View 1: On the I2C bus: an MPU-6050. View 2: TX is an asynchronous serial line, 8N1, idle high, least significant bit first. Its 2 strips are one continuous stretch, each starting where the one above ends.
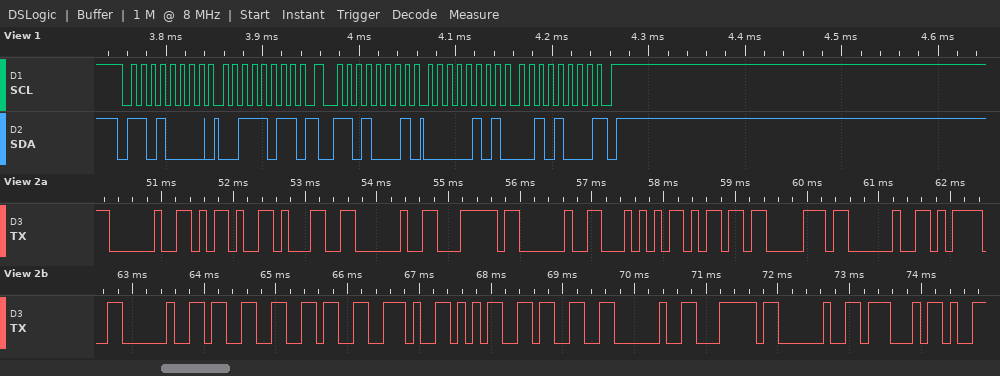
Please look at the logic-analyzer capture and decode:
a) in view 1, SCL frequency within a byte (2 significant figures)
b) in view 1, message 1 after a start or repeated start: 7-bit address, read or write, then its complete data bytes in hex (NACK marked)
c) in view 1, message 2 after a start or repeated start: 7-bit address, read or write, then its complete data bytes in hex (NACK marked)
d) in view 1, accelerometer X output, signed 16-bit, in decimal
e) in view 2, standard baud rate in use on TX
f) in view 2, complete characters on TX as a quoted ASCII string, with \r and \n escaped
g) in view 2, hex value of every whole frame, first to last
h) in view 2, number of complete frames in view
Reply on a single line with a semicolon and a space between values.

100 kHz; 0x68 write: 3B; 0x68 read: 05 28 NACK; 1320; 9600 baud; " -1 | Tmp = 36.53 | G"; 20 2D 31 20 7C 20 54 6D 70 20 3D 20 33 36 2E 35 33 20 7C 20 47; 21
